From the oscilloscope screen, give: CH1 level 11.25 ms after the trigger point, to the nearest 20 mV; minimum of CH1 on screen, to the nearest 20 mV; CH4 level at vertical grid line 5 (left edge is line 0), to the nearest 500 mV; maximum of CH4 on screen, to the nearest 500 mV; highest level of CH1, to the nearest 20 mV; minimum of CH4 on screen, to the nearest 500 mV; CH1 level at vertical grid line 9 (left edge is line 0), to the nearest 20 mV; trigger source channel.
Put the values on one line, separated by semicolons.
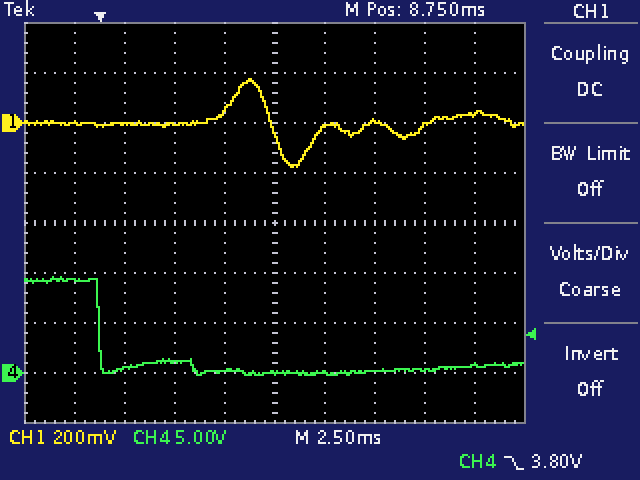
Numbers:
-20 mV; -180 mV; 0.0 V; 9.5 V; 180 mV; 0.0 V; 40 mV; CH4
